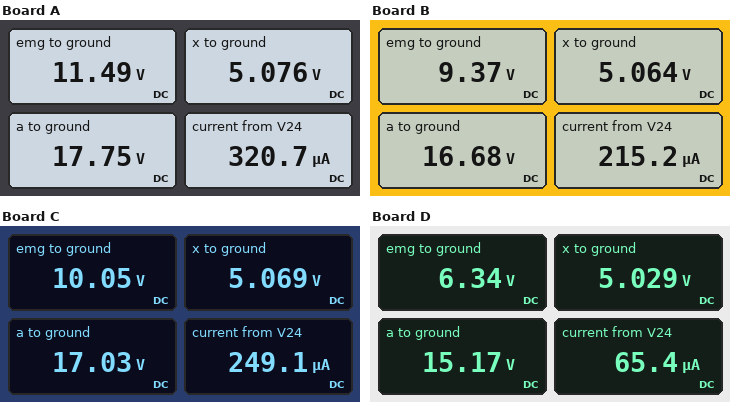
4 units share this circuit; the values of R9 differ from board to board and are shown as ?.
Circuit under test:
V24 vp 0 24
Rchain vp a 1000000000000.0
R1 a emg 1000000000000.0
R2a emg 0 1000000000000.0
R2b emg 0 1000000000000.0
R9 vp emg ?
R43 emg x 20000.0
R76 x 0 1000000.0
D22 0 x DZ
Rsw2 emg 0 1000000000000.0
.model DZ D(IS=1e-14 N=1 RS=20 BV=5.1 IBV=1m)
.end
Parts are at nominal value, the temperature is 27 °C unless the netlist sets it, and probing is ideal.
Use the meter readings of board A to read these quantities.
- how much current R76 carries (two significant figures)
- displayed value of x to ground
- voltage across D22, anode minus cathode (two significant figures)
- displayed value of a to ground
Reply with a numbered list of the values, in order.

1. 5.1 µA
2. 5.076 V
3. -5.1 V
4. 17.75 V
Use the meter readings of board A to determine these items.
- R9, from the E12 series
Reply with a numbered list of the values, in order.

1. 39 kΩ
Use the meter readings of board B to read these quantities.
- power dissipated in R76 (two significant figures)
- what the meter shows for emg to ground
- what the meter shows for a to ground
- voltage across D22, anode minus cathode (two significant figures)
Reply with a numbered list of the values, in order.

1. 26 µW
2. 9.37 V
3. 16.68 V
4. -5.1 V
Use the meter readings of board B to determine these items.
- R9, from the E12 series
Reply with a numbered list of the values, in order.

1. 68 kΩ
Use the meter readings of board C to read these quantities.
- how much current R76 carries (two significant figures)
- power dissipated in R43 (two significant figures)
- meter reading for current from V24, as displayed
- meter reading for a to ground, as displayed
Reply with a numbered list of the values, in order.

1. 5.1 µA
2. 1.2 mW
3. 249.1 µA
4. 17.03 V
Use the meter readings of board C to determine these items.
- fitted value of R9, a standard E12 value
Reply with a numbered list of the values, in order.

1. 56 kΩ
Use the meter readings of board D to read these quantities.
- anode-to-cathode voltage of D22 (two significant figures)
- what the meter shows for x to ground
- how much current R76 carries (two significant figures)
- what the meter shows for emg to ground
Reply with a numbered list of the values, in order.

1. -5.0 V
2. 5.029 V
3. 5.0 µA
4. 6.34 V
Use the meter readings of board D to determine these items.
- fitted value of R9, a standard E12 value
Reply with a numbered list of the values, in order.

1. 270 kΩ
